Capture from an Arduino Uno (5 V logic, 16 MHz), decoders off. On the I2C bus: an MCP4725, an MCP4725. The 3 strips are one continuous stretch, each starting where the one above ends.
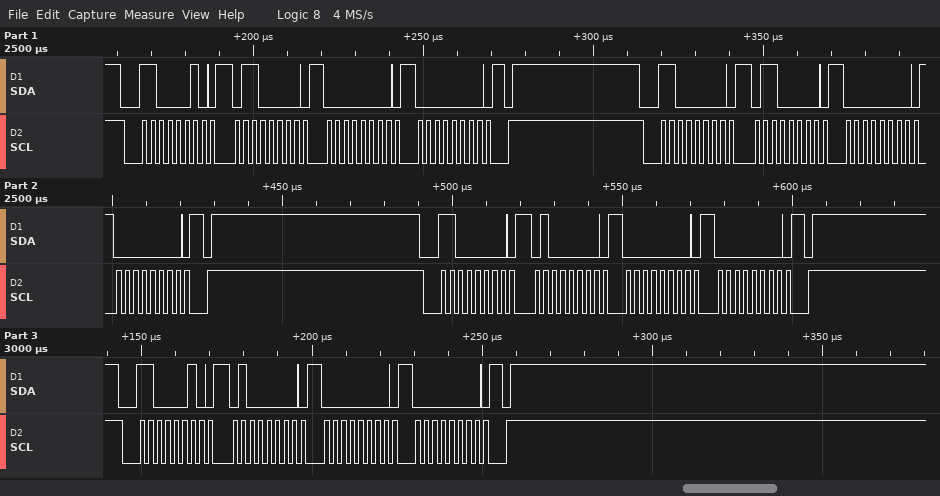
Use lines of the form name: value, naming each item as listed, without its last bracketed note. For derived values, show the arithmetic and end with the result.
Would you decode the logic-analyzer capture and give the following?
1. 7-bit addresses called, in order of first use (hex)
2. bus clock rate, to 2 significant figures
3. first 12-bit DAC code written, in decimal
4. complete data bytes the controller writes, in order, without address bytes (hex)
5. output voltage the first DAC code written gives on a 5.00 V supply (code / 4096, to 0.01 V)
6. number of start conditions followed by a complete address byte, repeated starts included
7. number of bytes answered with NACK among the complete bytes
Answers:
7-bit addresses called, in order of first use: 0x61 0x60
bus clock rate, to 2 significant figures: 400 kHz
first 12-bit DAC code written, in decimal: 0
complete data bytes the controller writes, in order, without address bytes: 60 00 00 60 00 00 40 00 00 40 00 00
output voltage the first DAC code written gives on a 5.00 V supply: 0 / 4096 x 5.00 V = 0.00 V
number of start conditions followed by a complete address byte, repeated starts included: 4
number of bytes answered with NACK among the complete bytes: 0
